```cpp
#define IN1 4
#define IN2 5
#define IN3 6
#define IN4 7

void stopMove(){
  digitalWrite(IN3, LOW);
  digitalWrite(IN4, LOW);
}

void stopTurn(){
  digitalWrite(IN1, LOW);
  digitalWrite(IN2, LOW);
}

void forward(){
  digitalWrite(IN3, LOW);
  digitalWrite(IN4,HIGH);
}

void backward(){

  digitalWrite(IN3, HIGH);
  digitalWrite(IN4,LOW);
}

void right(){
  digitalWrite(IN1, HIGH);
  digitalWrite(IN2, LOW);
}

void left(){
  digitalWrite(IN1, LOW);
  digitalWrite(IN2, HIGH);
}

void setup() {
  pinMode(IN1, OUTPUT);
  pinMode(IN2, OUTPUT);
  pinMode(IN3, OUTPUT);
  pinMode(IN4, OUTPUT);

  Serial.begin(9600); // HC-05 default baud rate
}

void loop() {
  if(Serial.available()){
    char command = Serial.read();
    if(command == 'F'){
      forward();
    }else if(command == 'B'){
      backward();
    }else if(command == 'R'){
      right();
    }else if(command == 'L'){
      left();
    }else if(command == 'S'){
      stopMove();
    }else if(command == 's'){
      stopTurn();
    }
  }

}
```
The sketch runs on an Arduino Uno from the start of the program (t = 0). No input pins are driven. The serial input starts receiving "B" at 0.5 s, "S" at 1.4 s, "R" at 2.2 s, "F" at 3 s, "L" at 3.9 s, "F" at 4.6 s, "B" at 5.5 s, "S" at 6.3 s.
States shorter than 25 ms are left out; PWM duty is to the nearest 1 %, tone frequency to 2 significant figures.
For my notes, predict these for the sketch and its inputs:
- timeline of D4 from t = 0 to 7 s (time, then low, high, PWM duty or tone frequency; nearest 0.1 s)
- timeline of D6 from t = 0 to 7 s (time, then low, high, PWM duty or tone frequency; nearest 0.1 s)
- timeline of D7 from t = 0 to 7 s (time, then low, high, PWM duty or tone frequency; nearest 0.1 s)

0 s low; 2.2 s high; 3.9 s low
0 s low; 0.5 s high; 1.4 s low; 5.5 s high; 6.3 s low
0 s low; 3 s high; 5.5 s low
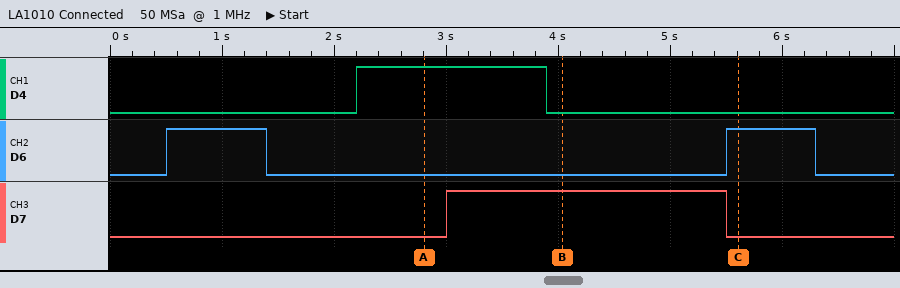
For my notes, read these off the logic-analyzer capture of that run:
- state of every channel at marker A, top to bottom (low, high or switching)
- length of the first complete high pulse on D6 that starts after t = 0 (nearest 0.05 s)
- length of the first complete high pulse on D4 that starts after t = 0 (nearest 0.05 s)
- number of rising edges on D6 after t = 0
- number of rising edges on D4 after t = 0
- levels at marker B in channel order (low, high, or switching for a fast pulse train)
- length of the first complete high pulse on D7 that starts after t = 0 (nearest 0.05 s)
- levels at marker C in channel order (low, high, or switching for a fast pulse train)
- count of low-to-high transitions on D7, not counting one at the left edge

D4 high, D6 low, D7 low
0.90 s
1.70 s
2
1
D4 low, D6 low, D7 high
2.50 s
D4 low, D6 high, D7 low
1
